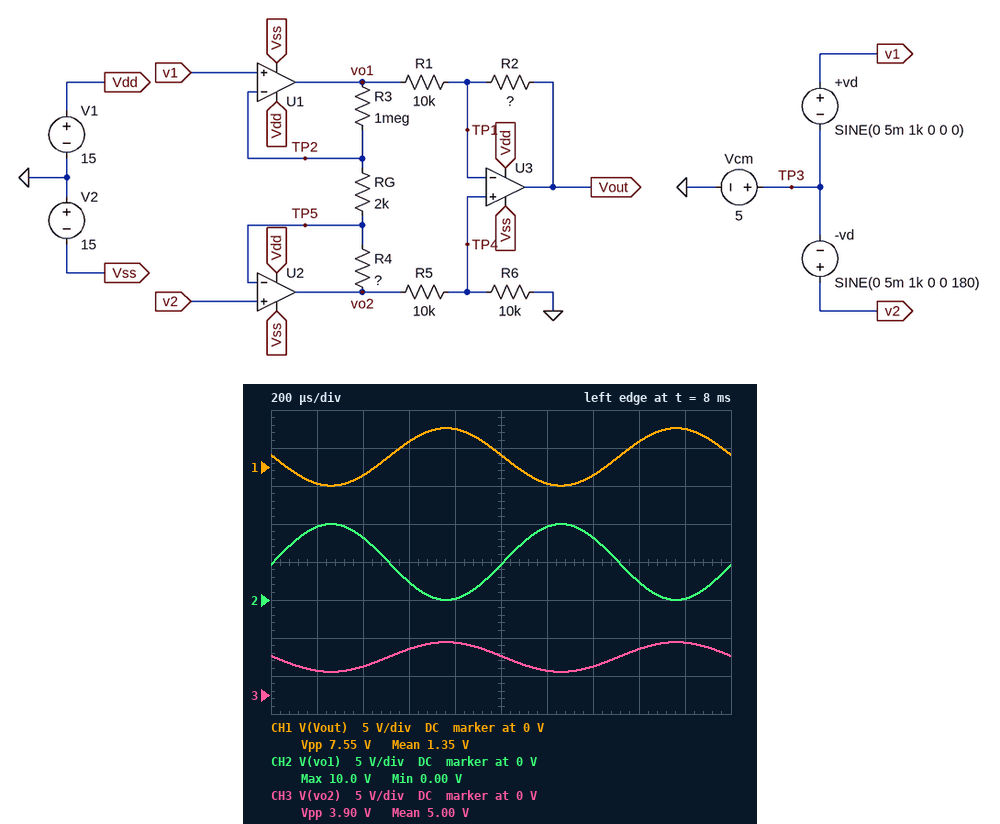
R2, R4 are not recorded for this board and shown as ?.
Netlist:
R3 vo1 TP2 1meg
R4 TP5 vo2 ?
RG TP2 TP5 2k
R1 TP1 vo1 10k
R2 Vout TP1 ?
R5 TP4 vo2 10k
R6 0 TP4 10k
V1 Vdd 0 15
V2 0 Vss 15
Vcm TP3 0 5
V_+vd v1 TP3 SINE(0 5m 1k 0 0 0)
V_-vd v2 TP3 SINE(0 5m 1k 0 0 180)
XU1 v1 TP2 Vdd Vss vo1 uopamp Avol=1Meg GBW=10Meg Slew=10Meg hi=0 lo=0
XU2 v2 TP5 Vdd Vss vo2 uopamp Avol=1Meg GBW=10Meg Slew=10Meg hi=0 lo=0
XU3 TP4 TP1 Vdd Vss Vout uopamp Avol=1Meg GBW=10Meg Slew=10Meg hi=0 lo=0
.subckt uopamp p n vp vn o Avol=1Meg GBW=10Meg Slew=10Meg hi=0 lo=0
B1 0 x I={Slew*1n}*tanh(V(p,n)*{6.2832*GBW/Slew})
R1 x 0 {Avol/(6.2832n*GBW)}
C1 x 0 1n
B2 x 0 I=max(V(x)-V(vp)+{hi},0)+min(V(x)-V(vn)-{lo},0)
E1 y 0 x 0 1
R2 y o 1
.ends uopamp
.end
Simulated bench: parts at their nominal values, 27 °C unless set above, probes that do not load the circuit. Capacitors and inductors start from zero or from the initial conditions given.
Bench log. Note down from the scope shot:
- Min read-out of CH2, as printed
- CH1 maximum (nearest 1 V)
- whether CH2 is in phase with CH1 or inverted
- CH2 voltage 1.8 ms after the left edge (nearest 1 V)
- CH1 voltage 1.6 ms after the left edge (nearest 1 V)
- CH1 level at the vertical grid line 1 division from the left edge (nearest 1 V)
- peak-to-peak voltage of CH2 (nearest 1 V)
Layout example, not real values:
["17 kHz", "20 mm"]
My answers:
["0.00 V", "5 V", "inverted", "0 V", "3 V", "-2 V", "10 V"]
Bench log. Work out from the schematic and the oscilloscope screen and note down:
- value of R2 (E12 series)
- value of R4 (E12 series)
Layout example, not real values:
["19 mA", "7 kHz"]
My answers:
["4.7 kΩ", "390 kΩ"]
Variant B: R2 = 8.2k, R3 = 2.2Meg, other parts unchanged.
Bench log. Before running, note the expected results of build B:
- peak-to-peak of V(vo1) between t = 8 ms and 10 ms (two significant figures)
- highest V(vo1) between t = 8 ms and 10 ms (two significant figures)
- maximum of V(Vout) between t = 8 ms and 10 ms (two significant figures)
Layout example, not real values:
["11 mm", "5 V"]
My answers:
["21 V", "15 V", "11 V"]
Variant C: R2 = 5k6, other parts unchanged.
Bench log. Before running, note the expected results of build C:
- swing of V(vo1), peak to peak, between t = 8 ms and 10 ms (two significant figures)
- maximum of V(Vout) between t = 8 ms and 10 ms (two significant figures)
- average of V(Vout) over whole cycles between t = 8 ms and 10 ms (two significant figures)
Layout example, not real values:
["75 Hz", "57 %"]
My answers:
["10 V", "5.4 V", "1.1 V"]
